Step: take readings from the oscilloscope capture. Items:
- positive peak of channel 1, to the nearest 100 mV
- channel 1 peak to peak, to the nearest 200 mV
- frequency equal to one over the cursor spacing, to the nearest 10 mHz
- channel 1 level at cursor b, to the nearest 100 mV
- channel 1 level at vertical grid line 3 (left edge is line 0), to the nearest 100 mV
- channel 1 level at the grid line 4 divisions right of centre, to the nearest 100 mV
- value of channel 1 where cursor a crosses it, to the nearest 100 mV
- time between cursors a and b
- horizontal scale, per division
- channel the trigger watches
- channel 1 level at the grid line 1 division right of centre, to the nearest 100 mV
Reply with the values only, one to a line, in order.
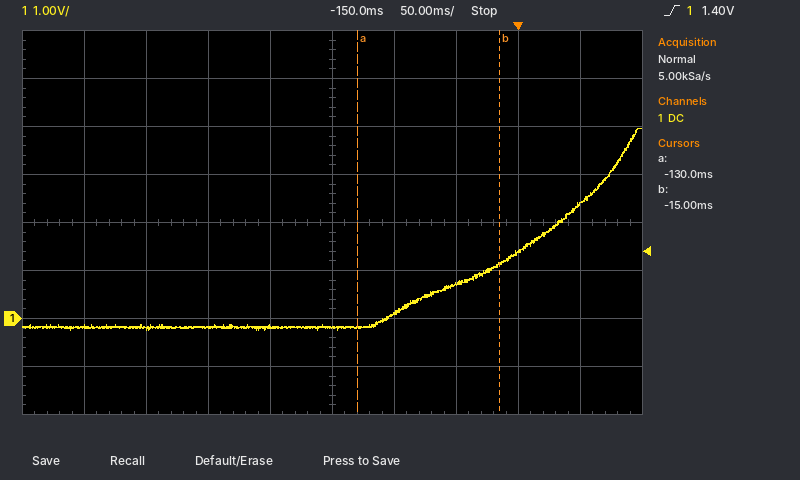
4.0 V
4.2 V
8.70 Hz
1.1 V
-200 mV
2.4 V
-200 mV
115 ms
50 ms
channel 1
100 mV
